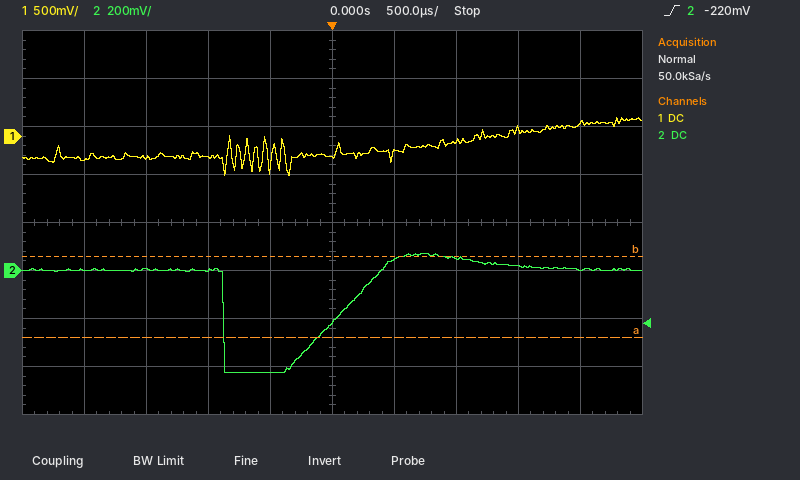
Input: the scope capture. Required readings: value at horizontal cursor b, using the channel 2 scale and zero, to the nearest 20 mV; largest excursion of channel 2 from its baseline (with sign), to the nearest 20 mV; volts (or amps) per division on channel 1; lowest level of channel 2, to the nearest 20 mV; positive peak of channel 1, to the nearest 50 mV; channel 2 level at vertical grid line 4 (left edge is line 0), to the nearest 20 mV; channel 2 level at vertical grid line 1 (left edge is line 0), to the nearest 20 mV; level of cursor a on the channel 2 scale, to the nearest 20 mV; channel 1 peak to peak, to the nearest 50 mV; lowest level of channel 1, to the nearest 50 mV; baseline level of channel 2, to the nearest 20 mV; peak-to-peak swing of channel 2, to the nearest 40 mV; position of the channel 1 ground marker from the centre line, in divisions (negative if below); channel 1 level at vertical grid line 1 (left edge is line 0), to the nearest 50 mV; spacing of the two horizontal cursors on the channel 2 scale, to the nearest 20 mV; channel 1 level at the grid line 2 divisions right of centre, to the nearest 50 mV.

60 mV
-420 mV
500 mV
-420 mV
200 mV
-420 mV
0 mV
-280 mV
600 mV
-400 mV
0 mV
480 mV
+1.8 div
-250 mV
340 mV
-50 mV
